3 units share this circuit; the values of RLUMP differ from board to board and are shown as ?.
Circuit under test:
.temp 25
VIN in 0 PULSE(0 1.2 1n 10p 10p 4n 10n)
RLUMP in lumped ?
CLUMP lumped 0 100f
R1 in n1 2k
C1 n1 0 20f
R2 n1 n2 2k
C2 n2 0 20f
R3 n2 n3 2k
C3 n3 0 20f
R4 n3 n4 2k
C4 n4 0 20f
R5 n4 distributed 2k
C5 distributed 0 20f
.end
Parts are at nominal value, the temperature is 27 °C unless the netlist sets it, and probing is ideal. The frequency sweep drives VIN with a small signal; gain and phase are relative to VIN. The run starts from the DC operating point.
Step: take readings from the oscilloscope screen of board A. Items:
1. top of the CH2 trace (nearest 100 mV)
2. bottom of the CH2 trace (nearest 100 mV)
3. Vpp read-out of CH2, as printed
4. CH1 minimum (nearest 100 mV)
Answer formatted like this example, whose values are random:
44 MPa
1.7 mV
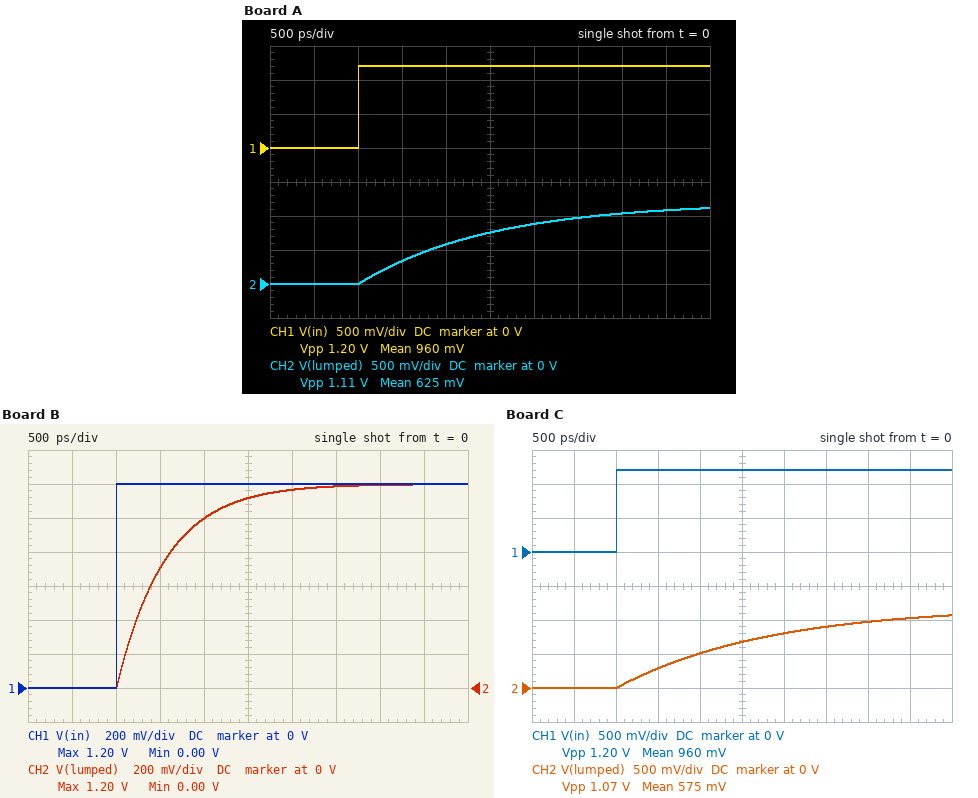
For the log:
1.1 V
0 V
1.11 V
0 V
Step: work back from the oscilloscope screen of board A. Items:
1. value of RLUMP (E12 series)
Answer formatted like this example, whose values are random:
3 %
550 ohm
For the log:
15 kΩ
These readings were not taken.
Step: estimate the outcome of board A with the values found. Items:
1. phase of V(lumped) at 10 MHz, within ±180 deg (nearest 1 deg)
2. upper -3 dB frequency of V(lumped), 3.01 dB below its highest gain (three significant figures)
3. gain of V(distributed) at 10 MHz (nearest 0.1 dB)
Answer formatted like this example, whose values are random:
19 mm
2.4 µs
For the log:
-5 deg
106 MHz
0 dB
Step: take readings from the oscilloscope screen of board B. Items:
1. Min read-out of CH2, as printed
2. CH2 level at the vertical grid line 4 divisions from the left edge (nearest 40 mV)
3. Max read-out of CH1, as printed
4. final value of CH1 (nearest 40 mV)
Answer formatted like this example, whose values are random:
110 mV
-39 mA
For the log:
0.00 V
1.00 V
1.20 V
1.20 V
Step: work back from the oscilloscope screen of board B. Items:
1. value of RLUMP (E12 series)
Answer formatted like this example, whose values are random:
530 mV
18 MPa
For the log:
5.6 kΩ
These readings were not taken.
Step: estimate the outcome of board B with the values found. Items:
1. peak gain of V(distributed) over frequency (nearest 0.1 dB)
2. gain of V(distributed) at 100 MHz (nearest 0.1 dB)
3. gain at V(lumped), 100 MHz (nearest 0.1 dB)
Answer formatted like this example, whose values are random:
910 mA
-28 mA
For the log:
0 dB
-0.4 dB
-0.5 dB
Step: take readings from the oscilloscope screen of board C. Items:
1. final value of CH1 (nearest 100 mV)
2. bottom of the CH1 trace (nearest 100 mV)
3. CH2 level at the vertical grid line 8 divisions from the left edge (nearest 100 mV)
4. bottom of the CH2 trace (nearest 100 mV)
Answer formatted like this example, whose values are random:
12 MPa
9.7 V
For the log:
1.2 V
0 V
1.0 V
0 V
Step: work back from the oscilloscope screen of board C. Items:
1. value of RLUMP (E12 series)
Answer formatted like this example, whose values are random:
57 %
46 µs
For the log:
18 kΩ
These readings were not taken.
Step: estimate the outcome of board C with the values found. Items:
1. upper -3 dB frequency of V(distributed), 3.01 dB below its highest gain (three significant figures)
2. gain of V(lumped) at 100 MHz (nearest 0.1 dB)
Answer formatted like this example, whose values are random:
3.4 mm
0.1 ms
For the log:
317 MHz
-3.6 dB
